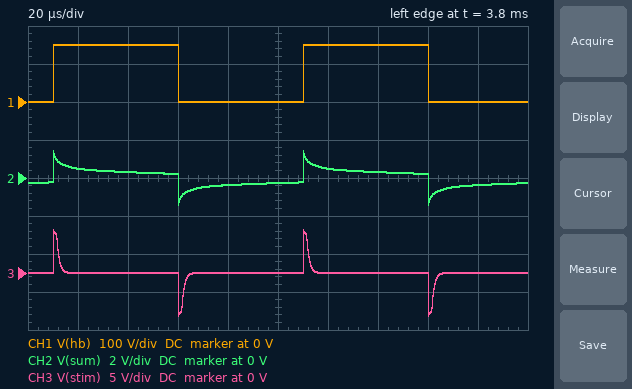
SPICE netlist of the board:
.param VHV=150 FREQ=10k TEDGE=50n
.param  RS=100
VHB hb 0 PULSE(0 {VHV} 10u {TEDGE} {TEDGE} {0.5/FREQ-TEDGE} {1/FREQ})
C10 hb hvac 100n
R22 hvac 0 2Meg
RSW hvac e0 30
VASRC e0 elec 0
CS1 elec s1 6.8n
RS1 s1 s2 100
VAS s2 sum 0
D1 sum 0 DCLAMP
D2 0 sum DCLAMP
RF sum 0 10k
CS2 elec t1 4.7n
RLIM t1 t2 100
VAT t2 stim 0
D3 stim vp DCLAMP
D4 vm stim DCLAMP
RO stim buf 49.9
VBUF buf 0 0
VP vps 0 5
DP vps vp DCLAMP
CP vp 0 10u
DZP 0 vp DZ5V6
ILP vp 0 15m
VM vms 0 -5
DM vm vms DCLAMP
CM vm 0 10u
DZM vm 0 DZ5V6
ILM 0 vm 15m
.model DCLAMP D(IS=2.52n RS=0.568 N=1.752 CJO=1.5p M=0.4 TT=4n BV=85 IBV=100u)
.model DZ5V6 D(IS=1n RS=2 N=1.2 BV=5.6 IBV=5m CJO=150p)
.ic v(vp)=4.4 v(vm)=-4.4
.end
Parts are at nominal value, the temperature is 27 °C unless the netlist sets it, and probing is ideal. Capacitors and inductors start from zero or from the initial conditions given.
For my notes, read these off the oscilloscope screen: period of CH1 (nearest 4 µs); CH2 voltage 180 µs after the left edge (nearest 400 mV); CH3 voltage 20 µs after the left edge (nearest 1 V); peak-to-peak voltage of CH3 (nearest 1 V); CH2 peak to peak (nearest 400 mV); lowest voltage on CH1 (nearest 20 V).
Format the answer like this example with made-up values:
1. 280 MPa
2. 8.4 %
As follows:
1. 100 µs
2. -400 mV
3. 0 V
4. 11 V
5. 2.8 V
6. 0 V
